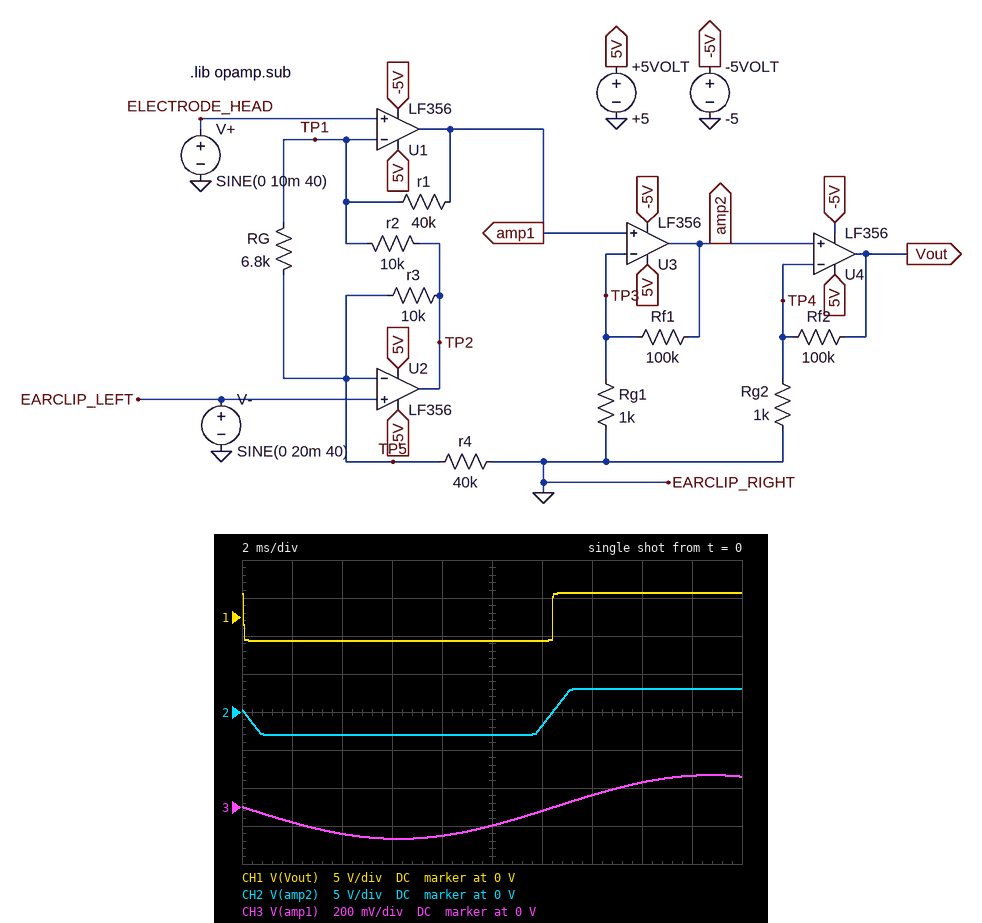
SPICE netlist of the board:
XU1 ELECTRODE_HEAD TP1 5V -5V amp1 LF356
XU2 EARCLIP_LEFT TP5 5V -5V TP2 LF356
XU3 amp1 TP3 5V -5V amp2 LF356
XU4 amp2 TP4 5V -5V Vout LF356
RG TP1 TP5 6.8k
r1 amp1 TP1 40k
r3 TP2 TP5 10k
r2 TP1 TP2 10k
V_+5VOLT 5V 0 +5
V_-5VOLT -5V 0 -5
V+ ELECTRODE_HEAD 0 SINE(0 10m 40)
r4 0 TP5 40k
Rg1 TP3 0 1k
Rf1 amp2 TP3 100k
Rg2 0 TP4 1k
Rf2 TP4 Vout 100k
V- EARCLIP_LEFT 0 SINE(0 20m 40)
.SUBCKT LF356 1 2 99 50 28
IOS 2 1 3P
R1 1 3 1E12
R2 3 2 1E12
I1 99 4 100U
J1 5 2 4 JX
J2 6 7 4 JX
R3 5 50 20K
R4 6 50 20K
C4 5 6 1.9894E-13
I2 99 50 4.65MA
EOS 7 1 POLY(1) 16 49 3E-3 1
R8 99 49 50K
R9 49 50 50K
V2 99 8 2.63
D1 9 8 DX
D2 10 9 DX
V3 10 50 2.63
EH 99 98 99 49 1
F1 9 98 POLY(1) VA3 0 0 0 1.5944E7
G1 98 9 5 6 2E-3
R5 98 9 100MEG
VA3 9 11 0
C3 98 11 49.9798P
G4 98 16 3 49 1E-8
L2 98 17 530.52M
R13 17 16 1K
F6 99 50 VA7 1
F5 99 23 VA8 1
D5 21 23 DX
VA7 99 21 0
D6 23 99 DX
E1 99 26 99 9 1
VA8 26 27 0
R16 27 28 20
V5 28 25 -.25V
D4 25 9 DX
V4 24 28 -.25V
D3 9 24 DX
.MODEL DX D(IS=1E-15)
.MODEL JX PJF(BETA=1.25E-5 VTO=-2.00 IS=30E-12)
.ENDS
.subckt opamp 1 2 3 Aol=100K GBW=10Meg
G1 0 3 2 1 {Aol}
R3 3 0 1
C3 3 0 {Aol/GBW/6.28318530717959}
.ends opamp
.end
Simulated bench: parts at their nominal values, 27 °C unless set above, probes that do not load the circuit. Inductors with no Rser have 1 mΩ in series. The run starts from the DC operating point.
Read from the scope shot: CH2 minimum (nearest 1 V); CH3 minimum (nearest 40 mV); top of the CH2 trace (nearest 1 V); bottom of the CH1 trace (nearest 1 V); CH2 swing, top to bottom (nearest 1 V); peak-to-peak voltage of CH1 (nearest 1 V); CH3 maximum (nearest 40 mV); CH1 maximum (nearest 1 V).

-3 V
-160 mV
3 V
-3 V
6 V
6 V
160 mV
3 V
